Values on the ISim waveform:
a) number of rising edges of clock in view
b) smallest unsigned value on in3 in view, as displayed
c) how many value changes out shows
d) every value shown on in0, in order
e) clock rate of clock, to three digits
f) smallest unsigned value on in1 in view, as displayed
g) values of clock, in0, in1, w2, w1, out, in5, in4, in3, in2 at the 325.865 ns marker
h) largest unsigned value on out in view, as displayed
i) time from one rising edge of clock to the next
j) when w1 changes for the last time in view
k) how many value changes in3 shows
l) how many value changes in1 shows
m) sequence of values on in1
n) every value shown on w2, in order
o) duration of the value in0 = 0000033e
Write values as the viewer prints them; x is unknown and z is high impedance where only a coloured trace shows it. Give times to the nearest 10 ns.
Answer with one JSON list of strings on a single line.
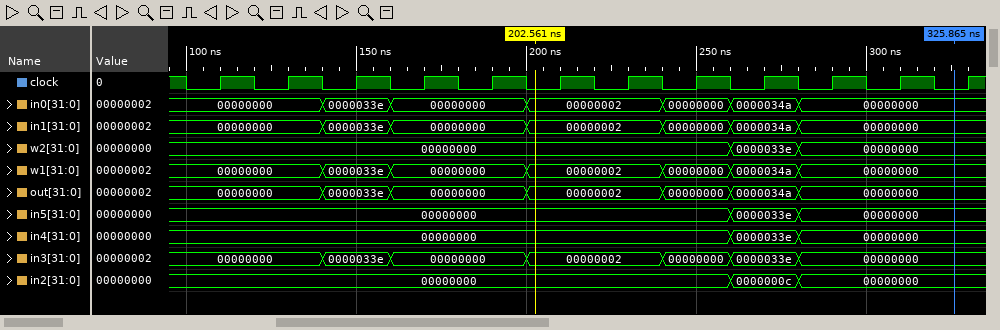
["12", "00000000", "6", "00000000, 0000033e, 00000000, 00000002, 00000000, 0000034a, 00000000", "50.0 MHz", "00000000", "clock=0, in0=00000000, in1=00000000, w2=00000000, w1=00000000, out=00000000, in5=00000000, in4=00000000, in3=00000000, in2=00000000", "0000034a", "20 ns", "280 ns", "6", "6", "00000000, 0000033e, 00000000, 00000002, 00000000, 0000034a, 00000000", "00000000, 0000033e, 00000000", "20 ns"]
